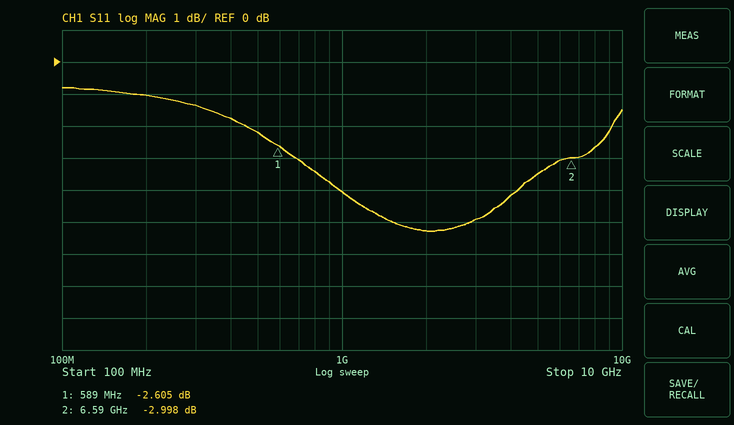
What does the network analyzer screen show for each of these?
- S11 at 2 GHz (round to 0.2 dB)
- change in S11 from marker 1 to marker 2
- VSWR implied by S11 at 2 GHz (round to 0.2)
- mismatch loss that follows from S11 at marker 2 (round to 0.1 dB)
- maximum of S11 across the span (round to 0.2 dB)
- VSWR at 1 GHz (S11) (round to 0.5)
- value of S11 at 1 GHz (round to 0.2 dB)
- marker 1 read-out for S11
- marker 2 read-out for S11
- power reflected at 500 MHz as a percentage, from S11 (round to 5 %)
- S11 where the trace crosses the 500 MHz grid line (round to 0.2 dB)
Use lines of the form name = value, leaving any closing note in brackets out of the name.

S11 at 2 GHz = -5.2 dB
change in S11 from marker 1 to marker 2 = -0.393 dB
VSWR implied by S11 at 2 GHz = 3.4
mismatch loss that follows from S11 at marker 2 = 3.0 dB
maximum of S11 across the span = -0.8 dB
VSWR at 1 GHz (S11) = 4.5
value of S11 at 1 GHz = -4.0 dB
marker 1 read-out for S11 = -2.605 dB
marker 2 read-out for S11 = -2.998 dB
power reflected at 500 MHz as a percentage, from S11 = 60 %
S11 where the trace crosses the 500 MHz grid line = -2.2 dB
